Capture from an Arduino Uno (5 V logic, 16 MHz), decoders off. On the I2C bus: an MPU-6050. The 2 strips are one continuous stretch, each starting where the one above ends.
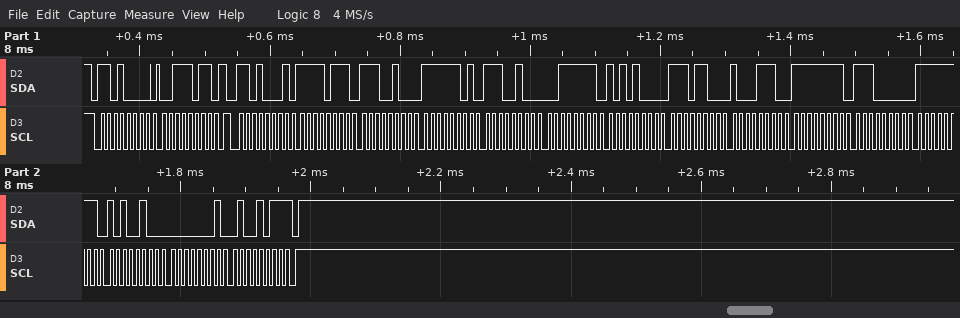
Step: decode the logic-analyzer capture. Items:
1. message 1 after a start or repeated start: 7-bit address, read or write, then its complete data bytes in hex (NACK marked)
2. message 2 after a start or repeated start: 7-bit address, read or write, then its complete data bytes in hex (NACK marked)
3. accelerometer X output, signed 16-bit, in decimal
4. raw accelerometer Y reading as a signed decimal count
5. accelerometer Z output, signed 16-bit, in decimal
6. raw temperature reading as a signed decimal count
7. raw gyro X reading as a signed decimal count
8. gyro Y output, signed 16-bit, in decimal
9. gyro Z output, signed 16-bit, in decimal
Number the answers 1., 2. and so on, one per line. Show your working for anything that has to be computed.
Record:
1. 0x68 write: 3B
2. 0x68 read: F7 E4 FD E4 3F A8 EC 8E FF E0 FF A4 01 4B NACK
3. 0xF7E4 = -2076
4. 0xFDE4 = -540
5. 0x3FA8 = 16296
6. 0xEC8E = -4978
7. 0xFFE0 = -32
8. 0xFFA4 = -92
9. 0x014B = 331
